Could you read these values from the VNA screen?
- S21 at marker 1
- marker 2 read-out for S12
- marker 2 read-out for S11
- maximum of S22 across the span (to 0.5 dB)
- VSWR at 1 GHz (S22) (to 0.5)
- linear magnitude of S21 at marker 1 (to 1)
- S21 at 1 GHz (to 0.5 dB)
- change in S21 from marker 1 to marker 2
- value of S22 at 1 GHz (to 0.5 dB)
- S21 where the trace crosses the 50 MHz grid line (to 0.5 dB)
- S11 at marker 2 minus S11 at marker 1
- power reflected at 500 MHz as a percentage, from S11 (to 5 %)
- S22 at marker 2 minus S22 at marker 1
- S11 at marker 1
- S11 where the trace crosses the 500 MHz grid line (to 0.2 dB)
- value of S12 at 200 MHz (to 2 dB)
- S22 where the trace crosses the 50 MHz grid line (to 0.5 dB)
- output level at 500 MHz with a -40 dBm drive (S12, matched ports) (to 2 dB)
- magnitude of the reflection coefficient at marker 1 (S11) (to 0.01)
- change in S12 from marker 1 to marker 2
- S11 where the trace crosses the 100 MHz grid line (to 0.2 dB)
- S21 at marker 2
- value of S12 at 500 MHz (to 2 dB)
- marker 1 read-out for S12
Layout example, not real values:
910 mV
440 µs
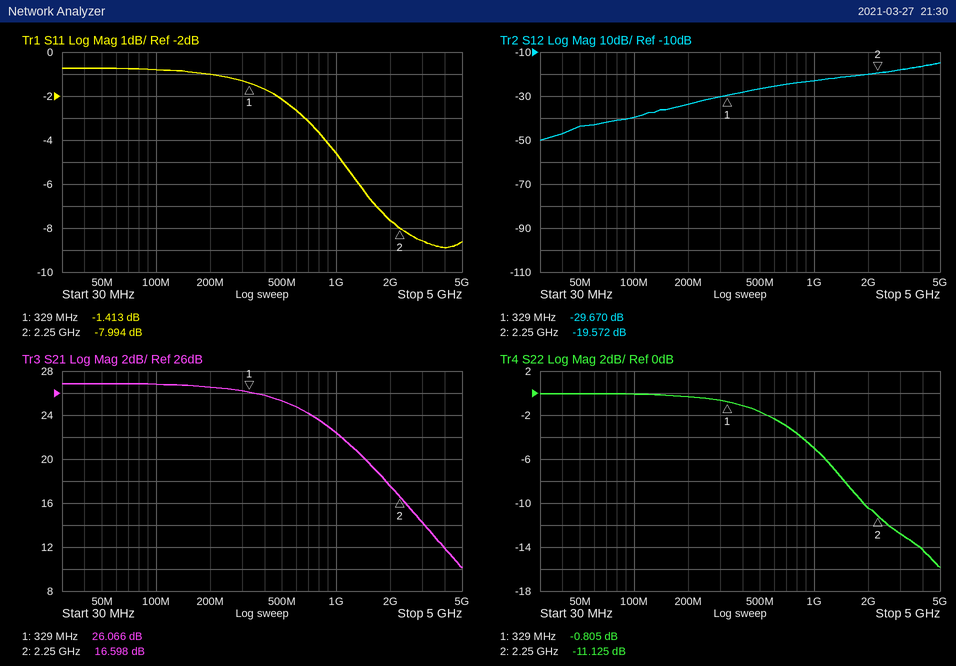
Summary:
26.066 dB
-19.572 dB
-7.994 dB
0.0 dB
3.5
20
22.5 dB
-9.468 dB
-5.0 dB
27.0 dB
-6.581 dB
60 %
-10.320 dB
-1.413 dB
-2.2 dB
-34 dB
0.0 dB
-66 dBm
0.85
10.098 dB
-0.8 dB
16.598 dB
-26 dB
-29.670 dB
